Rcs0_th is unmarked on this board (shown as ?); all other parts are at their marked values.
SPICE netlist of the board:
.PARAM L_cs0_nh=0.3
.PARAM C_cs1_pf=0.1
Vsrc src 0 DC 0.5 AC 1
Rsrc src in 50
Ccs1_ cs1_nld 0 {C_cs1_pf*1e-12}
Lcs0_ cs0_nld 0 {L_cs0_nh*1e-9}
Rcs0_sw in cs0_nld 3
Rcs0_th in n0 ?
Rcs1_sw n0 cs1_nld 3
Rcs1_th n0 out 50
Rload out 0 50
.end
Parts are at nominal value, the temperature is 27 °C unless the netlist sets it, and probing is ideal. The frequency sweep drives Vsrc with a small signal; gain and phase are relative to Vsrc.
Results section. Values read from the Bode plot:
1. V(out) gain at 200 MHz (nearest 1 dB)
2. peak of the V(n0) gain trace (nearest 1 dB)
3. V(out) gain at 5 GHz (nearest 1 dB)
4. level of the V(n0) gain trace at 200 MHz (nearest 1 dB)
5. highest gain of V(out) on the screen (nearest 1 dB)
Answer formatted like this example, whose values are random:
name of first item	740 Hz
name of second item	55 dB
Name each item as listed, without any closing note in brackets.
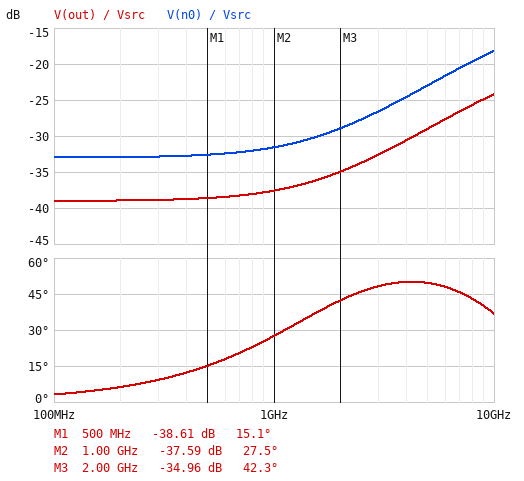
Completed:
V(out) gain at 200 MHz	-39 dB
peak of the V(n0) gain trace	-18 dB
V(out) gain at 5 GHz	-29 dB
level of the V(n0) gain trace at 200 MHz	-33 dB
highest gain of V(out) on the screen	-24 dB
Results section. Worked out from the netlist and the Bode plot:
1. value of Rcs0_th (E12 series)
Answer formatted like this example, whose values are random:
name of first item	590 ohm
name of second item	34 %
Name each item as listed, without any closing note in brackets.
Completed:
value of Rcs0_th	150 Ω
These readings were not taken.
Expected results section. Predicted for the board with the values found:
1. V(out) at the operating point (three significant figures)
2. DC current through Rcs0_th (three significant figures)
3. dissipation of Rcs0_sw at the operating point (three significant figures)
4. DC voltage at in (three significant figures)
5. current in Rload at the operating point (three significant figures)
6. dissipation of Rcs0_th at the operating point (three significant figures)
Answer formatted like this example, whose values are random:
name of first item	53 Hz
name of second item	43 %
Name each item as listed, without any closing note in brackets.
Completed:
V(out) at the operating point	5.60 mV
DC current through Rcs0_th	112 µA
dissipation of Rcs0_sw at the operating point	261 µW
DC voltage at in	28.0 mV
current in Rload at the operating point	112 µA
dissipation of Rcs0_th at the operating point	1.88 µW
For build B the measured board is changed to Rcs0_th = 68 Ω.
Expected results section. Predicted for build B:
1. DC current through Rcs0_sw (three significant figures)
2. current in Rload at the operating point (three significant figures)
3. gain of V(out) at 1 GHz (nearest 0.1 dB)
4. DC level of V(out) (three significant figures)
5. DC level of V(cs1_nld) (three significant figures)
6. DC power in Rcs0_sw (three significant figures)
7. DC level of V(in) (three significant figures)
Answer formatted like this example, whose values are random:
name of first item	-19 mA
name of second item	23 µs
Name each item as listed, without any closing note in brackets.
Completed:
DC current through Rcs0_sw	9.28 mA
current in Rload at the operating point	166 µA
gain of V(out) at 1 GHz	-34.2 dB
DC level of V(out)	8.28 mV
DC level of V(cs1_nld)	16.6 mV
DC power in Rcs0_sw	258 µW
DC level of V(in)	27.8 mV
